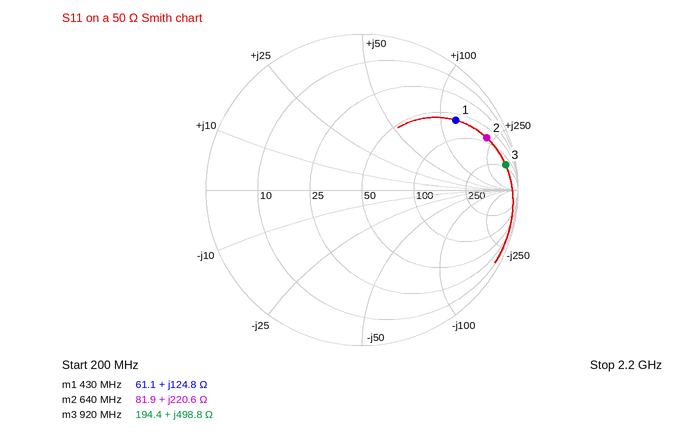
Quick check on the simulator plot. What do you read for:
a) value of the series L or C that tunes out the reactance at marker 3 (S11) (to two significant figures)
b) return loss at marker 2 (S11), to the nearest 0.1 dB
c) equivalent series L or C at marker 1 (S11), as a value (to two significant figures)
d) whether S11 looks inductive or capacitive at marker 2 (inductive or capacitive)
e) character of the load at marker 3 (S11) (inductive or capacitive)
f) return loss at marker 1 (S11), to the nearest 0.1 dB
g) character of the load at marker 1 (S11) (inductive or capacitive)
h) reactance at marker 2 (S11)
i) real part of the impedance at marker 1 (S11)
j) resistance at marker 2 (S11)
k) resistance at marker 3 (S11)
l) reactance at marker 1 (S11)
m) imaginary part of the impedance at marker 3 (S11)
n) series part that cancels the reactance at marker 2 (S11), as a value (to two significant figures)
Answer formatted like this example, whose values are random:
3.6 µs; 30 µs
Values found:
350 fF; 1.2 dB; 46 nH; inductive; inductive; 2.5 dB; inductive; +220.6 Ω; 61.1 Ω; 81.9 Ω; 194.4 Ω; +124.8 Ω; +498.8 Ω; 1.1 pF
